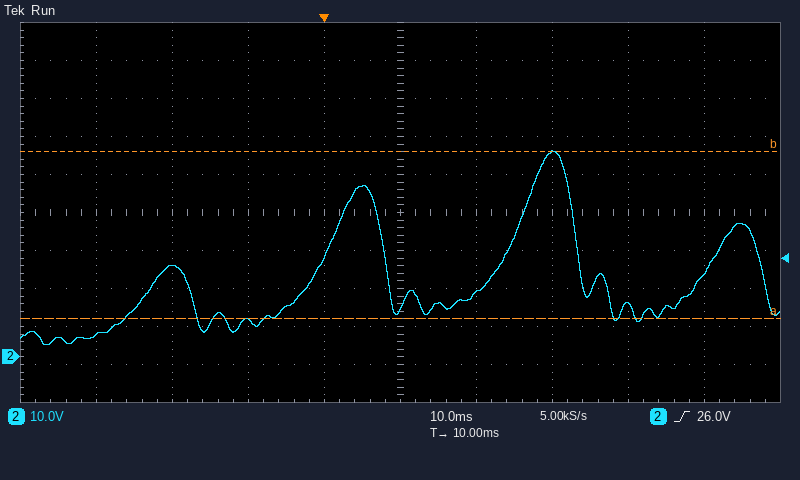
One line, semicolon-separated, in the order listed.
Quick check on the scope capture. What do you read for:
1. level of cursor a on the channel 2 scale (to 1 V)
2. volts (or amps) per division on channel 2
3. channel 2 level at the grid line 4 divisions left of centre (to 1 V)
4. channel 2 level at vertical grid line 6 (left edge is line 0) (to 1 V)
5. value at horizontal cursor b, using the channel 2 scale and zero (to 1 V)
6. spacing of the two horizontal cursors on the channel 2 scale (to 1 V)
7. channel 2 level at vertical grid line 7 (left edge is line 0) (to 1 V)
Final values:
10 V; 10 V; 6 V; 17 V; 54 V; 44 V; 54 V
